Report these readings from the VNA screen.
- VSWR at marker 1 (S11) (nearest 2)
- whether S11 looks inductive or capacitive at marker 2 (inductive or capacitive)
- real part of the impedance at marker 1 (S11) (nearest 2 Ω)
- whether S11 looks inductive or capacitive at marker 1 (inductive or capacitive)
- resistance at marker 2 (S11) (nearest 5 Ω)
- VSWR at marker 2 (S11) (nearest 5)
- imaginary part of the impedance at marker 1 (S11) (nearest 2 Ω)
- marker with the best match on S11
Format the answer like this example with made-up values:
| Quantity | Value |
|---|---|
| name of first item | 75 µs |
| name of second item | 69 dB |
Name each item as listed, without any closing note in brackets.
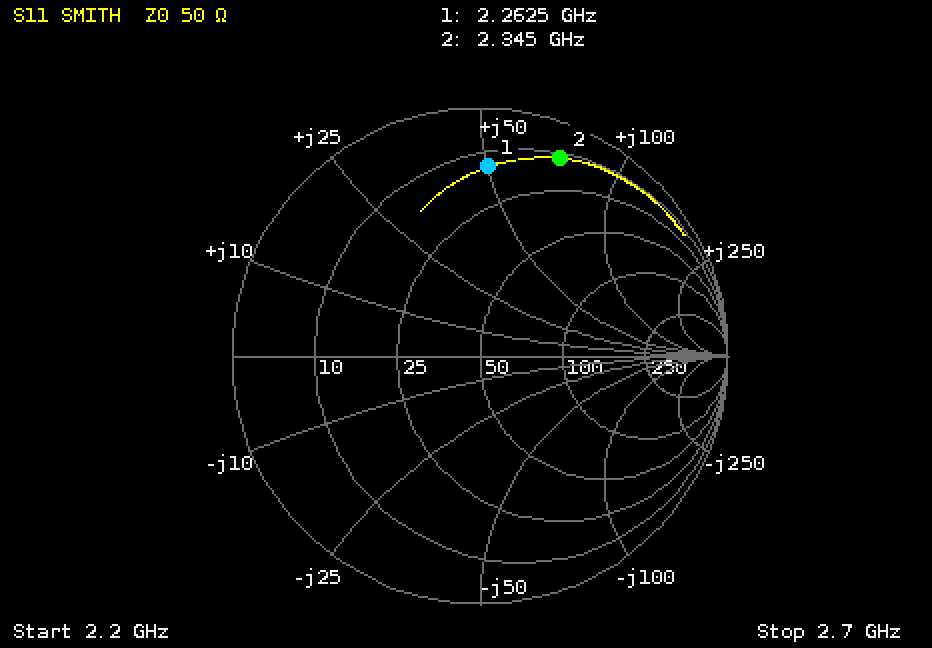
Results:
| Quantity | Value |
|---|---|
| VSWR at marker 1 (S11) | 8 |
| whether S11 looks inductive or capacitive at marker 2 | inductive |
| real part of the impedance at marker 1 (S11) | 14 Ω |
| whether S11 looks inductive or capacitive at marker 1 | inductive |
| resistance at marker 2 (S11) | 10 Ω |
| VSWR at marker 2 (S11) | 15 |
| imaginary part of the impedance at marker 1 (S11) | +50 Ω |
| marker with the best match on S11 | marker 1 |
